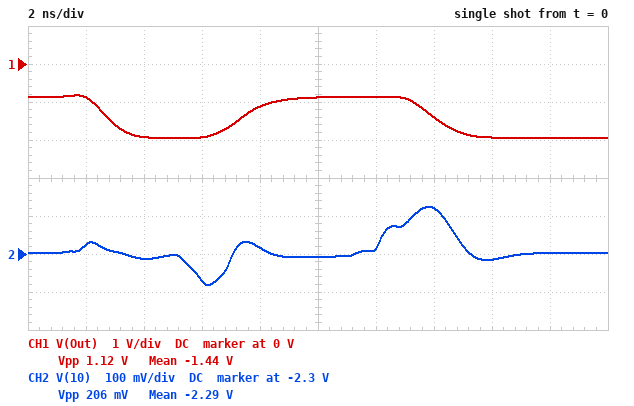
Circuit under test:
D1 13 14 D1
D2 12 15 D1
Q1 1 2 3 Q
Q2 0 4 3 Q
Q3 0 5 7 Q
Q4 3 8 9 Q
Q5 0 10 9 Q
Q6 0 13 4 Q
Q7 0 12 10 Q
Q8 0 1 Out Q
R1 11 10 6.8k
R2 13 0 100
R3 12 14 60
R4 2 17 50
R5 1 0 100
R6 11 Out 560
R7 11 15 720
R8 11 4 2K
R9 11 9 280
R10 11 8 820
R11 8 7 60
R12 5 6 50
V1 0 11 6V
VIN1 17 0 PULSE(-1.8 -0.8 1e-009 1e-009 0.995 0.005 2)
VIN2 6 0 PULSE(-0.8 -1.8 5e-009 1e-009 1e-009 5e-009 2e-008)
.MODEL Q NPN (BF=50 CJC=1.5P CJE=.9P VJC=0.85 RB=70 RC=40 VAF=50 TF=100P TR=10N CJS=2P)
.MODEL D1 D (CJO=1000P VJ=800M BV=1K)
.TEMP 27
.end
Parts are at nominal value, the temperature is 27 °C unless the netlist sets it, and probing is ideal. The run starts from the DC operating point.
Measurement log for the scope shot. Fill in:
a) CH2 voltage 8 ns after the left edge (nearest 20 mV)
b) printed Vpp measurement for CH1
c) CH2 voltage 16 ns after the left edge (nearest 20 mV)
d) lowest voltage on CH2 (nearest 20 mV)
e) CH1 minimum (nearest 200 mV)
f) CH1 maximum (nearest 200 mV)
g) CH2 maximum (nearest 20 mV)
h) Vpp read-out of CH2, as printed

-2.28 V
1.12 V
-2.32 V
-2.38 V
-2.0 V
-800 mV
-2.18 V
206 mV
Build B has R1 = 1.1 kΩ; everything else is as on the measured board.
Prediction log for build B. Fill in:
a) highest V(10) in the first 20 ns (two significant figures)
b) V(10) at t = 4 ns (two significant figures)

-2.3 V
-2.4 V
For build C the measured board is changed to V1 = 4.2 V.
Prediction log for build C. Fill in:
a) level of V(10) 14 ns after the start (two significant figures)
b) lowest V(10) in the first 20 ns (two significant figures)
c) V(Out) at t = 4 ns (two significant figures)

-1.9 V
-2.0 V
-1.4 V
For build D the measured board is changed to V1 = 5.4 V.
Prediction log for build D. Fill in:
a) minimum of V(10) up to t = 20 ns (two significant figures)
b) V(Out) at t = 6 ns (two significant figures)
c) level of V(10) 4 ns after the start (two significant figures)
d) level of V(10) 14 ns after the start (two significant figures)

-2.3 V
-1.8 V
-2.2 V
-2.1 V
